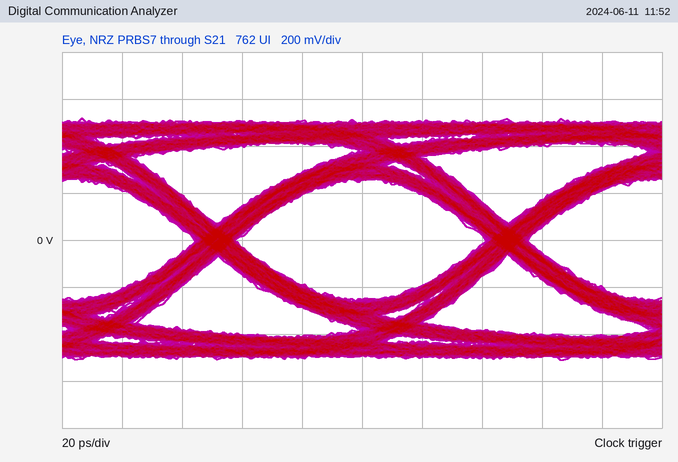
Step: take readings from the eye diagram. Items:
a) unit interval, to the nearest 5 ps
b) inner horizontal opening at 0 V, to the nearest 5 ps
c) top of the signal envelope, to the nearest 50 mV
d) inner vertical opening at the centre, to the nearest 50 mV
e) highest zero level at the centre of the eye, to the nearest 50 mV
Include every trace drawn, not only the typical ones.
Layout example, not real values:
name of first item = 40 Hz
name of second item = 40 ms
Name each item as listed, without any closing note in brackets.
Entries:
unit interval, to the nearest 5 ps = 95 ps
inner horizontal opening at 0 V, to the nearest 5 ps = 85 ps
top of the signal envelope, to the nearest 50 mV = 500 mV
inner vertical opening at the centre, to the nearest 50 mV = 500 mV
highest zero level at the centre of the eye, to the nearest 50 mV = -250 mV
